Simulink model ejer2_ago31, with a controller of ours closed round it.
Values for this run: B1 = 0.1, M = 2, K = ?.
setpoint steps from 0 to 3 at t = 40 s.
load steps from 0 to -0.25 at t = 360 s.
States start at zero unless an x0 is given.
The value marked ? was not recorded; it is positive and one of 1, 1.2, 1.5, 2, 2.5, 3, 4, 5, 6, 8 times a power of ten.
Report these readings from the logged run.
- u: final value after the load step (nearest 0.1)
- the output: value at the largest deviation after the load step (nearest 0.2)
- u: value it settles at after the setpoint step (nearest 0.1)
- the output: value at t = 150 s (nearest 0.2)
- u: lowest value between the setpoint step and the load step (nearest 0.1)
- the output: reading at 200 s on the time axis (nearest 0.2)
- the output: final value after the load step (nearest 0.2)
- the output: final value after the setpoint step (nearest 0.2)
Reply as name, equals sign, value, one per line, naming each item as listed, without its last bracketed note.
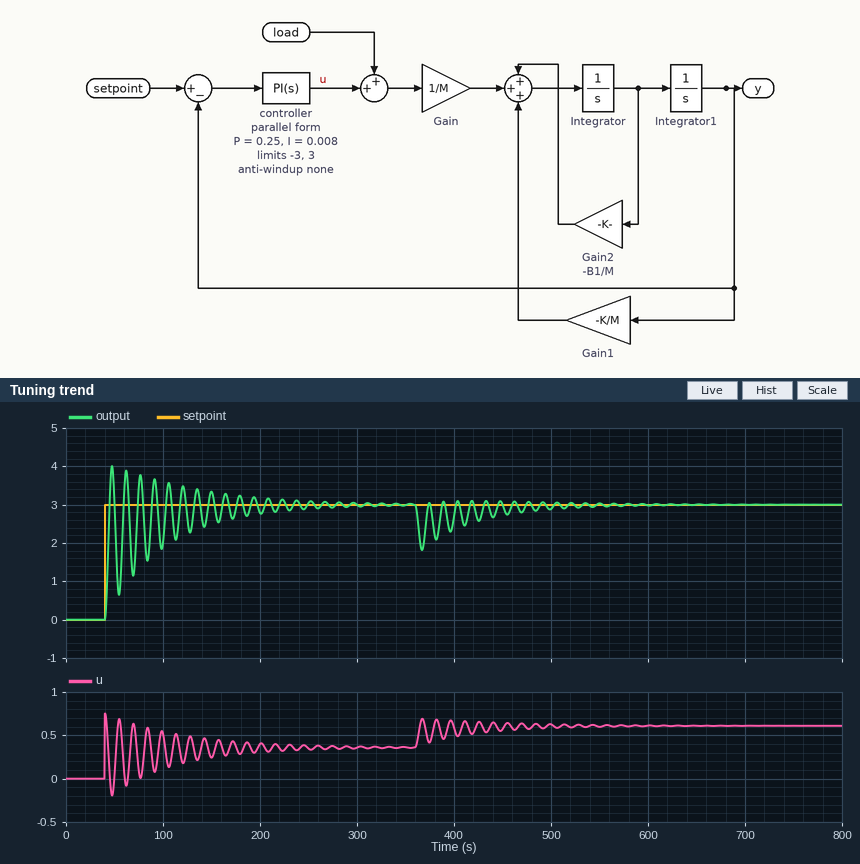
u: final value after the load step = 0.6
the output: value at the largest deviation after the load step = 1.8
u: value it settles at after the setpoint step = 0.4
the output: value at t = 150 s = 3.4
u: lowest value between the setpoint step and the load step = -0.2
the output: reading at 200 s on the time axis = 2.8
the output: final value after the load step = 3.0
the output: final value after the setpoint step = 3.0
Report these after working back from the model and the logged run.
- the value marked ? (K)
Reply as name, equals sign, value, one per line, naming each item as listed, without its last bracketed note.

the value marked ? = 0.12
